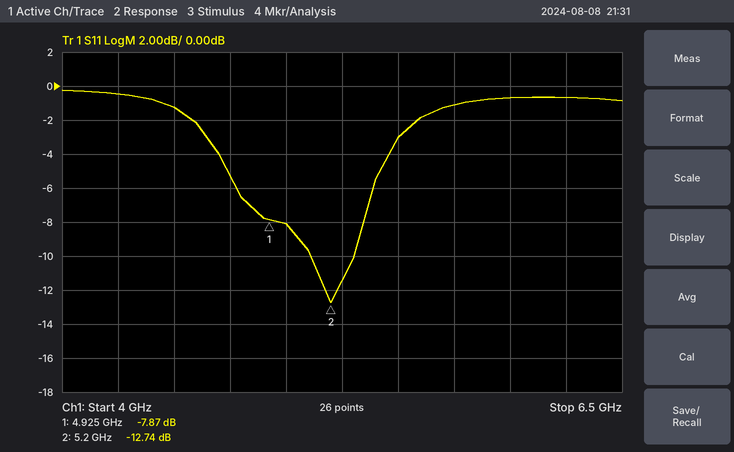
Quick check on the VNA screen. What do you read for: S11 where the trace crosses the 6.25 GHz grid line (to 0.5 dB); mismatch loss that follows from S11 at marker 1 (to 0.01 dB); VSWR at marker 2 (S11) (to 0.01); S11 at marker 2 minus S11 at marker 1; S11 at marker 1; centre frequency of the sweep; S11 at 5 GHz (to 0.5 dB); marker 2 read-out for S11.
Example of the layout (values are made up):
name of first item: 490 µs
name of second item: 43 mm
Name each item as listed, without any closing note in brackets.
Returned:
S11 where the trace crosses the 6.25 GHz grid line: -0.5 dB
mismatch loss that follows from S11 at marker 1: 0.77 dB
VSWR at marker 2 (S11): 1.60
S11 at marker 2 minus S11 at marker 1: -4.87 dB
S11 at marker 1: -7.87 dB
centre frequency of the sweep: 5.25 GHz
S11 at 5 GHz: -8.0 dB
marker 2 read-out for S11: -12.74 dB
